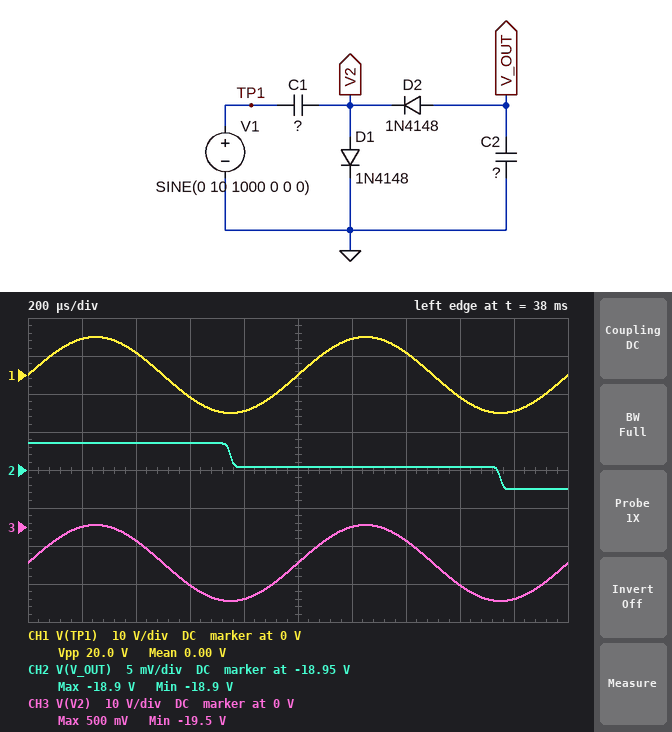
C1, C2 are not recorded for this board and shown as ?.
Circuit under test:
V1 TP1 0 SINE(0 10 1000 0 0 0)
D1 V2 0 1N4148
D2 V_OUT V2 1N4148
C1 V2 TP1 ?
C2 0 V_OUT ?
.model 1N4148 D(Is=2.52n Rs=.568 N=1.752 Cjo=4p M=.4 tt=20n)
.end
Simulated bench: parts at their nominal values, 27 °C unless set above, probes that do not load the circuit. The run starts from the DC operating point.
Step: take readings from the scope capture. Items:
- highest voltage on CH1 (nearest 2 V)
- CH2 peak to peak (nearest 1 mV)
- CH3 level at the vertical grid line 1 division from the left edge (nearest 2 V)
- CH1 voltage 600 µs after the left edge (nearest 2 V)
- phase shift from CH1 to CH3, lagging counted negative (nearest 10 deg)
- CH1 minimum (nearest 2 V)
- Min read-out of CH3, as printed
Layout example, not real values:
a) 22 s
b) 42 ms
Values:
a) 10 V
b) 6 mV
c) 0 V
d) -6 V
e) 0 deg
f) -10 V
g) -19.5 V
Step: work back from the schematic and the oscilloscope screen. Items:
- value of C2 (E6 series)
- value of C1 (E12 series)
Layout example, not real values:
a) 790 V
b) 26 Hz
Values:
a) 2.2 µF
b) 1.5 µF
